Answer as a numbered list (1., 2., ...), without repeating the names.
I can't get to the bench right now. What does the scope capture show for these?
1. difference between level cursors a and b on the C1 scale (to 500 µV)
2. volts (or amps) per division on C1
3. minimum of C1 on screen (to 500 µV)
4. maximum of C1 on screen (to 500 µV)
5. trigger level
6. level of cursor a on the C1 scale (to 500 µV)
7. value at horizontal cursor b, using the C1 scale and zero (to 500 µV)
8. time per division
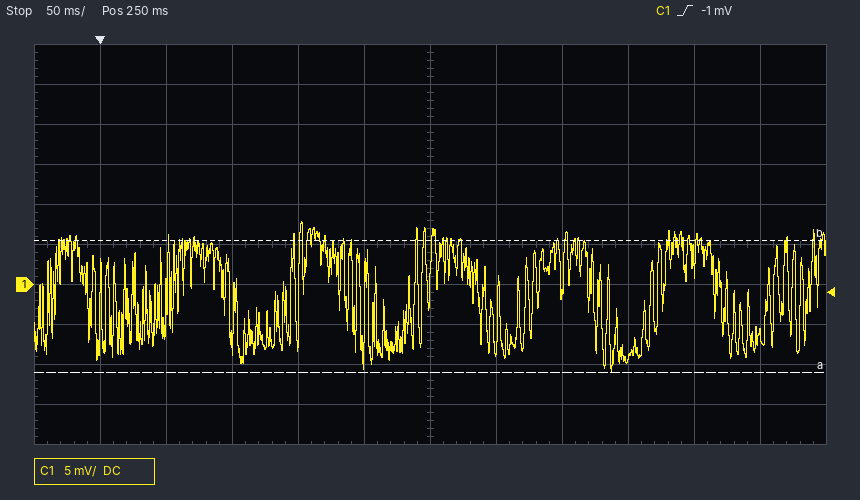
1. 16.5 mV
2. 5 mV
3. -11.0 mV
4. 8.0 mV
5. -1 mV
6. -11.0 mV
7. 5.5 mV
8. 50 ms
